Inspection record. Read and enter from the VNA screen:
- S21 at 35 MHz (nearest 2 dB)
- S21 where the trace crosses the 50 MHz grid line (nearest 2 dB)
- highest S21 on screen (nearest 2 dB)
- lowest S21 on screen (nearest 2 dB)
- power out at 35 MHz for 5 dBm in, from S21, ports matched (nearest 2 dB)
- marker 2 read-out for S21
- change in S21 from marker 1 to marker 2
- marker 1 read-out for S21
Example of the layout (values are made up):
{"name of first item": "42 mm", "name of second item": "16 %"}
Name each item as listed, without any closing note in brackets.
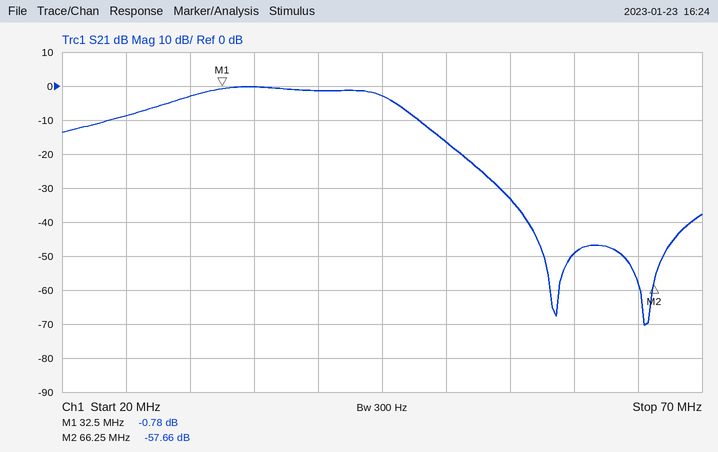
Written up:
{"S21 at 35 MHz": "0 dB", "S21 where the trace crosses the 50 MHz grid line": "-16 dB", "highest S21 on screen": "0 dB", "lowest S21 on screen": "-70 dB", "power out at 35 MHz for 5 dBm in, from S21, ports matched": "4 dBm", "marker 2 read-out for S21": "-57.66 dB", "change in S21 from marker 1 to marker 2": "-56.88 dB", "marker 1 read-out for S21": "-0.78 dB"}
